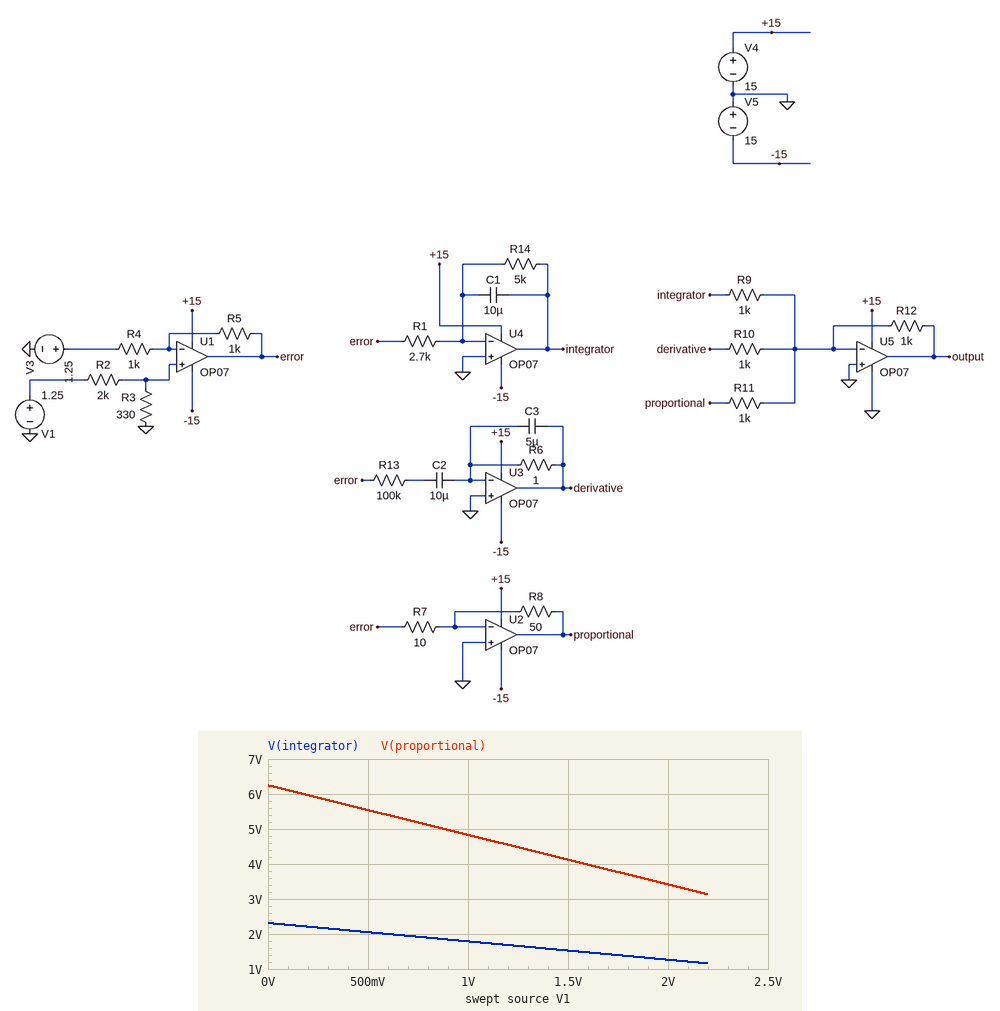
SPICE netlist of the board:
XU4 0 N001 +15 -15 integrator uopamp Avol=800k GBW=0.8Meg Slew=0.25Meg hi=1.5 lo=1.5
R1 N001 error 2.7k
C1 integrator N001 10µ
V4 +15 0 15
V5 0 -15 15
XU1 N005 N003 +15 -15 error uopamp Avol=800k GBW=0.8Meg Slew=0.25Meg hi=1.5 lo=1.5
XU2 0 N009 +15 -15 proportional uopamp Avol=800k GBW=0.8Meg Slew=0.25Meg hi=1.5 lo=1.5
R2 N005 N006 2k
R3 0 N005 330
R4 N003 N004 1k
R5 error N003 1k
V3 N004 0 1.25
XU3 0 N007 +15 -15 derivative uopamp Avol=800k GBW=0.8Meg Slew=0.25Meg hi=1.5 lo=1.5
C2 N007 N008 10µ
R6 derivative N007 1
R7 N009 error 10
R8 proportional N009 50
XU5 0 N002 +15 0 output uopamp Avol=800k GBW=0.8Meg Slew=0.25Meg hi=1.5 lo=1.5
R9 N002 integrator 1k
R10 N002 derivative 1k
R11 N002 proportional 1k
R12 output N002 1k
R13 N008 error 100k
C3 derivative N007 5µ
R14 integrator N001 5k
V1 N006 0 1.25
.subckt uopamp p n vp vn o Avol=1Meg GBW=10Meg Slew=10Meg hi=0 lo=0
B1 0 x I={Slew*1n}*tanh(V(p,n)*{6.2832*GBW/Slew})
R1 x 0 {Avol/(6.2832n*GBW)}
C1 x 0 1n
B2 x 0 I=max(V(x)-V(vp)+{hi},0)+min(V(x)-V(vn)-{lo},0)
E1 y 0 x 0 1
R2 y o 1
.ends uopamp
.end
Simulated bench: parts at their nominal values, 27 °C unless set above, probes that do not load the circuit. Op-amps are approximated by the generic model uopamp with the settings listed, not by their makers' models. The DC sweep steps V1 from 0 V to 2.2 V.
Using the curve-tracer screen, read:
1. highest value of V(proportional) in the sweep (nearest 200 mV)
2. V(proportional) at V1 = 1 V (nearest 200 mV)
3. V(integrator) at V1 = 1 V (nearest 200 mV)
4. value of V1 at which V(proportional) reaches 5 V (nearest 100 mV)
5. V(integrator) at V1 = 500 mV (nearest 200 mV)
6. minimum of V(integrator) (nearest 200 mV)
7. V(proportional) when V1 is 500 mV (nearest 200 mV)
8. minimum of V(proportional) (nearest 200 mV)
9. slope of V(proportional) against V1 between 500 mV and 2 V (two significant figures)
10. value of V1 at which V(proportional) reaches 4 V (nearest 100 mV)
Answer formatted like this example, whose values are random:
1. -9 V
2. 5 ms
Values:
1. 6.2 V
2. 4.8 V
3. 1.8 V
4. 900 mV
5. 2.0 V
6. 1.2 V
7. 5.6 V
8. 3.2 V
9. -1.4 V/V
10. 1.6 V
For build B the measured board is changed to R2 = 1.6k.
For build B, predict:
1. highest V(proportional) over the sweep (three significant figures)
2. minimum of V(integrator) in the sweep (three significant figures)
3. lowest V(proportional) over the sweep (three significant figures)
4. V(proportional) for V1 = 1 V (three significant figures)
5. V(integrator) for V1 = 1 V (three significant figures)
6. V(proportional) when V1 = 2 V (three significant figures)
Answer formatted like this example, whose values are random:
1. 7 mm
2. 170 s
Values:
1. 6.25 V
2. 922 mV
3. 2.49 V
4. 4.54 V
5. 1.68 V
6. 2.83 V
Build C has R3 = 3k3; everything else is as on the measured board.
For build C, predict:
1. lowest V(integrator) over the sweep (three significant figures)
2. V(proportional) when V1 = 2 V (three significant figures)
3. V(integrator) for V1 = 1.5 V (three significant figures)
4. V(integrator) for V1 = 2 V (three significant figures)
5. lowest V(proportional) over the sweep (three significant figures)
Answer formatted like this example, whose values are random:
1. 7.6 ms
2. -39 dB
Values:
1. -2.76 V
2. -6.20 V
3. -1.14 V
4. -2.30 V
5. -7.45 V
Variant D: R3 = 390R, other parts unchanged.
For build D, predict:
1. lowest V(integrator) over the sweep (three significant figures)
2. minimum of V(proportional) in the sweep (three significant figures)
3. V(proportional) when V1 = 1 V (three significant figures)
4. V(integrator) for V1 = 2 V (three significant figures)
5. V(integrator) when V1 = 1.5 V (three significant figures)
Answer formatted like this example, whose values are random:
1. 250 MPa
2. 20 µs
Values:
1. 985 mV
2. 2.66 V
3. 4.62 V
4. 1.11 V
5. 1.41 V
